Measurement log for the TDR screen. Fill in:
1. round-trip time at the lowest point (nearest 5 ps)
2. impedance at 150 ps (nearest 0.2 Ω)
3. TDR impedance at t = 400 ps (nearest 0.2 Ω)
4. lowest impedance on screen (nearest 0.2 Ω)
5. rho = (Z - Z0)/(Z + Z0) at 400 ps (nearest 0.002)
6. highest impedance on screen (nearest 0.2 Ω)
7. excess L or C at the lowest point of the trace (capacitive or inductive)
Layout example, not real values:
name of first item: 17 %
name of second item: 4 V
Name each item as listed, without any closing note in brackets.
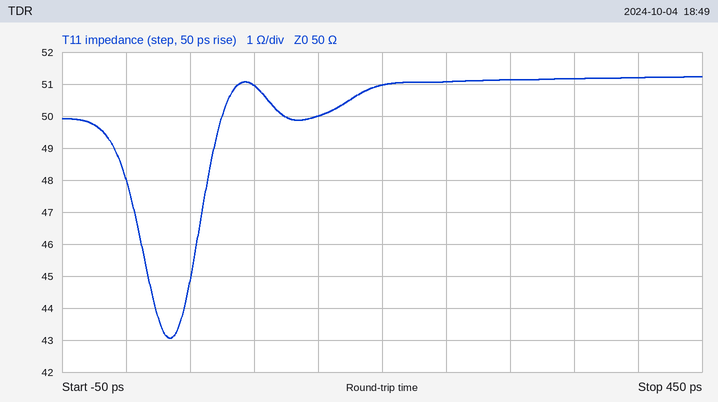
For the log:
round-trip time at the lowest point: 35 ps
impedance at 150 ps: 50.0 Ω
TDR impedance at t = 400 ps: 51.2 Ω
lowest impedance on screen: 43.0 Ω
rho = (Z - Z0)/(Z + Z0) at 400 ps: +0.012
highest impedance on screen: 51.2 Ω
excess L or C at the lowest point of the trace: capacitive
